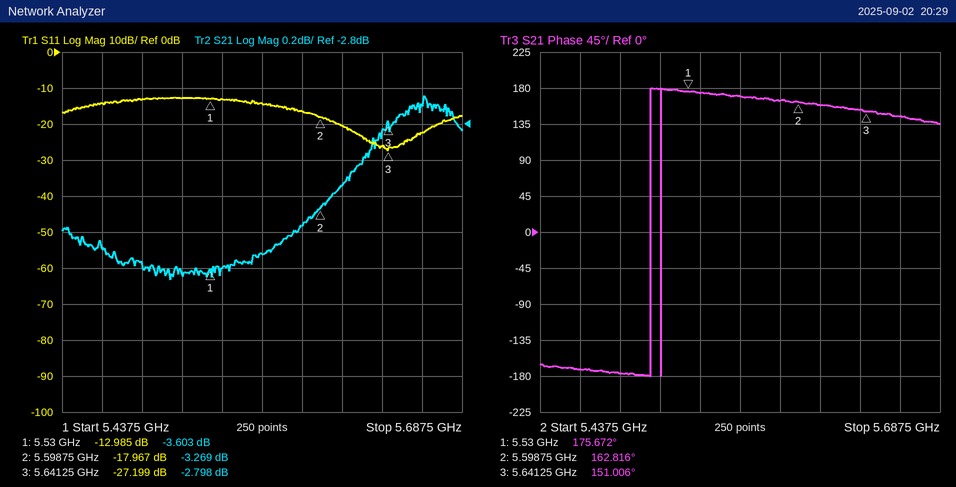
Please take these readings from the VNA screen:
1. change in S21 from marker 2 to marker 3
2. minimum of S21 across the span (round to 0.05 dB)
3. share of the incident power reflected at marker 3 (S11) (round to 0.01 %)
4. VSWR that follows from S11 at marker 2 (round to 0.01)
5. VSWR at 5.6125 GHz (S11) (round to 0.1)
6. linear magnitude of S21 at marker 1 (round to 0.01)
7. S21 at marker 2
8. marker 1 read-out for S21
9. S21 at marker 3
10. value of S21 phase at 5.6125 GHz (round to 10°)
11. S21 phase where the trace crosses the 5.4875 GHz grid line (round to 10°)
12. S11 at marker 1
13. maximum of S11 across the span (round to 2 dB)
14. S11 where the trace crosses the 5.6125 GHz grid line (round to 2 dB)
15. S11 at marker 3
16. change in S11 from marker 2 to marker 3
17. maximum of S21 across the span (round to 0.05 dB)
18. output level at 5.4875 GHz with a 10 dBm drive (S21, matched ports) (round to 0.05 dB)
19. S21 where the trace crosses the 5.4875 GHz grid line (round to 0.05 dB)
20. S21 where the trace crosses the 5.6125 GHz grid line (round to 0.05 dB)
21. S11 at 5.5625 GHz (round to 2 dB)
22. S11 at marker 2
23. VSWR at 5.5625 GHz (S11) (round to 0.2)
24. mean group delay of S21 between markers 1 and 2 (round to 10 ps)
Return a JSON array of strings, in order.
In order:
["0.471 dB", "-3.65 dB", "0.19 %", "1.29", "1.2", "0.66", "-3.269 dB", "-3.603 dB", "-2.798 dB", "160°", "-180°", "-12.985 dB", "-12 dB", "-20 dB", "-27.199 dB", "-9.232 dB", "-2.65 dB", "6.40 dBm", "-3.60 dB", "-3.15 dB", "-14 dB", "-17.967 dB", "1.4", "520 ps"]
